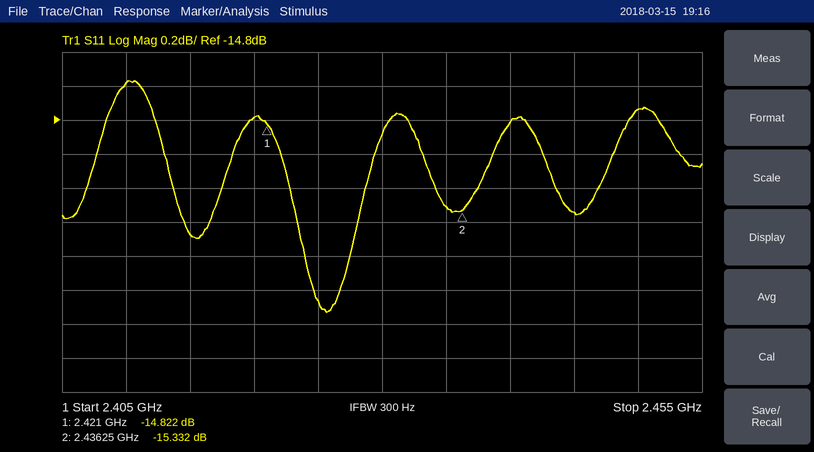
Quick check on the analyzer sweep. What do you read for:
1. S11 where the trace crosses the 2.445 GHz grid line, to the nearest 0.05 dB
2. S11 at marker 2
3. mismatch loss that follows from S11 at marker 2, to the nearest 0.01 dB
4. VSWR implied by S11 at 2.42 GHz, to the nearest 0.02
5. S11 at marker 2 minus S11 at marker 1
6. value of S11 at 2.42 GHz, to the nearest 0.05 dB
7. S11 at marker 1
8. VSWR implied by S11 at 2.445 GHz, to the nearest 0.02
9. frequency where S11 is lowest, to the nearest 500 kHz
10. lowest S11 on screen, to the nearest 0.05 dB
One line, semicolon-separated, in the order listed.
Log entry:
-15.35 dB; -15.332 dB; 0.13 dB; 1.44; -0.510 dB; -14.80 dB; -14.822 dB; 1.42; 2.4255 GHz; -15.95 dB
